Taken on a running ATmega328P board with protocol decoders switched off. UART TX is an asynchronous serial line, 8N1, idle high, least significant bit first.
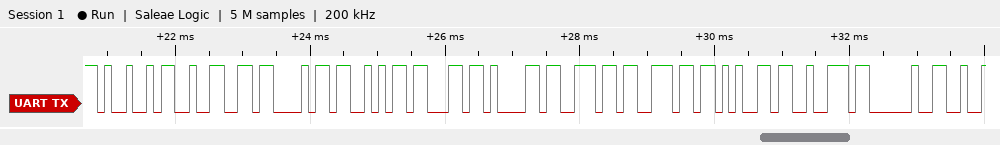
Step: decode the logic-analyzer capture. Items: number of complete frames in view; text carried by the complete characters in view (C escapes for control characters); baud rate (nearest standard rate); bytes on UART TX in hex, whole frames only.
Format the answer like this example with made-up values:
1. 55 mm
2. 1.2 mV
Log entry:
1. 11
2. "I2CScanner "
3. 9600 baud
4. 49 32 43 53 63 61 6E 6E 65 72 20
